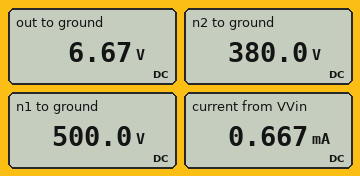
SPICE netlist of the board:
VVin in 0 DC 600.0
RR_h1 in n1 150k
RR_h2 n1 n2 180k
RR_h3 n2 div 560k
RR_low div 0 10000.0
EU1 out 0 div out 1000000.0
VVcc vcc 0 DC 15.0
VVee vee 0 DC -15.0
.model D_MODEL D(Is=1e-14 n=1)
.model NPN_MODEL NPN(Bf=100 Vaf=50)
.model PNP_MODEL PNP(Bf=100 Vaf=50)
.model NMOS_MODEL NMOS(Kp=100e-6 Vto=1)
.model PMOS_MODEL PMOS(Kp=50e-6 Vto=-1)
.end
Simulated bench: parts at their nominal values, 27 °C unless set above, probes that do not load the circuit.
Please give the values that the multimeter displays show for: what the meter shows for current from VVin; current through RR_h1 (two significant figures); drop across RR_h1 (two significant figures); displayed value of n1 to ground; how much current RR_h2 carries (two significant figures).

0.667 mA
670 µA
100 V
500.0 V
670 µA
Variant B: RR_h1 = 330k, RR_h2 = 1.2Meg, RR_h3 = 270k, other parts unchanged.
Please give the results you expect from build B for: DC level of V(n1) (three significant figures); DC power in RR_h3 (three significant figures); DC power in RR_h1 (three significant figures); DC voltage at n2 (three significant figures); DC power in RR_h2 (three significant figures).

491 V
29.7 mW
36.3 mW
92.8 V
132 mW
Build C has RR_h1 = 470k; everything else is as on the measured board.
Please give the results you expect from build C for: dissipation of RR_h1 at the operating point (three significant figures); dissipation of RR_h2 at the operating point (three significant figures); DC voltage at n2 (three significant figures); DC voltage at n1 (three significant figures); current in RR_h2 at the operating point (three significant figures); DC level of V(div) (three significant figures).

114 mW
43.5 mW
280 V
369 V
492 µA
4.92 V
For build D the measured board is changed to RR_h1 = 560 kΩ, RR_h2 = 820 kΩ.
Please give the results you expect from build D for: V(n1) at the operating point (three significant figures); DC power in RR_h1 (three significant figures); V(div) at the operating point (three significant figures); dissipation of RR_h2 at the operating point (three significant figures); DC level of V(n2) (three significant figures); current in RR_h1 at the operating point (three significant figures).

428 V
53.0 mW
3.08 V
77.6 mW
175 V
308 µA
